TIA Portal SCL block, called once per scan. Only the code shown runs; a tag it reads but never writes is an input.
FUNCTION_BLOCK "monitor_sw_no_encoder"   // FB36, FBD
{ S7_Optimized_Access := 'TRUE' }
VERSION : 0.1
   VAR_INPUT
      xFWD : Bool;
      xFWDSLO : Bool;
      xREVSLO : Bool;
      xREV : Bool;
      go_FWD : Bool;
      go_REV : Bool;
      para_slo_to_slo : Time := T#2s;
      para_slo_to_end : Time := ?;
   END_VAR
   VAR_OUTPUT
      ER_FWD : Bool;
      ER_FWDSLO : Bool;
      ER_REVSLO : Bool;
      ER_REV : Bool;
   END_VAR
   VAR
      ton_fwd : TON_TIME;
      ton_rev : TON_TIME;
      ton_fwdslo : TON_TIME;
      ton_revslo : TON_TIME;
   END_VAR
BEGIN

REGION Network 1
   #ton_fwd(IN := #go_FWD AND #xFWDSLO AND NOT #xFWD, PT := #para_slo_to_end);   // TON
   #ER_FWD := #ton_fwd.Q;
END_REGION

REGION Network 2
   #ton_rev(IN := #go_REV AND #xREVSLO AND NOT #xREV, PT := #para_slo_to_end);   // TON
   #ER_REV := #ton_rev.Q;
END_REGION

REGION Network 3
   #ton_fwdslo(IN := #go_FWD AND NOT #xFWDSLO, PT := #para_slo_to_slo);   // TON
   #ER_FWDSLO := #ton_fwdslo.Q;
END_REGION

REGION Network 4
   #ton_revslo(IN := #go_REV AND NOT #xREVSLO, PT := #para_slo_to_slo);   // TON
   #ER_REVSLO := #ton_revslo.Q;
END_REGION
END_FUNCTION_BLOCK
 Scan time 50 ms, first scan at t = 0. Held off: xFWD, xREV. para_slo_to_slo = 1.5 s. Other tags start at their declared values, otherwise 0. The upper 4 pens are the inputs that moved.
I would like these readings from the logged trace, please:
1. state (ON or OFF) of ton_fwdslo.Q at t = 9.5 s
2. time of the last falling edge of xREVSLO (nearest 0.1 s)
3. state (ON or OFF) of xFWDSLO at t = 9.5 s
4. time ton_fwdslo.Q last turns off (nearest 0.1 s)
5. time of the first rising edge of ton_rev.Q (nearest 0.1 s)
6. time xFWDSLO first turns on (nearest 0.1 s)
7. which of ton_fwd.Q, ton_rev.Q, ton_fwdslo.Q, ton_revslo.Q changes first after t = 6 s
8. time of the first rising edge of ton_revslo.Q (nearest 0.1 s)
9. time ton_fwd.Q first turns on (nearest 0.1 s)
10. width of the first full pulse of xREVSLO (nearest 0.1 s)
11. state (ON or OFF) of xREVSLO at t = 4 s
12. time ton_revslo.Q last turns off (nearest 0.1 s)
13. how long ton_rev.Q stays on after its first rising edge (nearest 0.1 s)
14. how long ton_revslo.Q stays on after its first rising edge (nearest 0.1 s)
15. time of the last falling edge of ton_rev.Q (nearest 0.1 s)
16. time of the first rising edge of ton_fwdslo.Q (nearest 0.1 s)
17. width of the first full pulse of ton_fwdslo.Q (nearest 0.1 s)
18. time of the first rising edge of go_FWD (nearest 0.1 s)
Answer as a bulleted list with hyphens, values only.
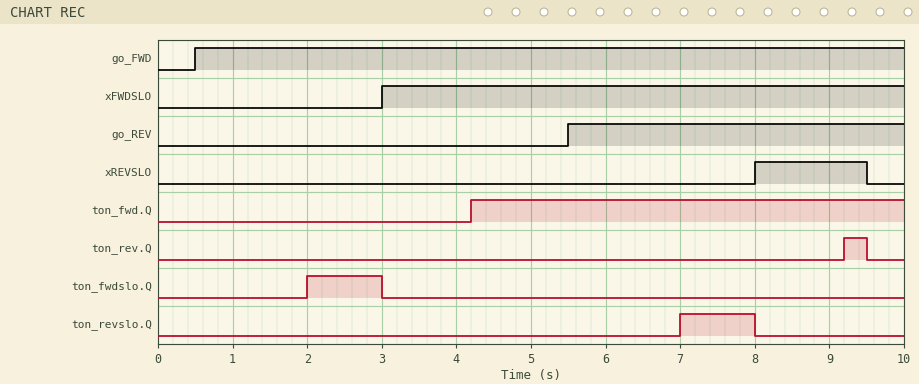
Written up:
- OFF
- 9.5 s
- ON
- 3.0 s
- 9.2 s
- 3.0 s
- ton_revslo.Q
- 7.0 s
- 4.2 s
- 1.5 s
- OFF
- 8.0 s
- 0.3 s
- 1.0 s
- 9.5 s
- 2.0 s
- 1.0 s
- 0.5 s
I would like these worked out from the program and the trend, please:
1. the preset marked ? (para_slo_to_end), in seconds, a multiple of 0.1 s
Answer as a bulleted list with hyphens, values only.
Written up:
- 1.2 s
